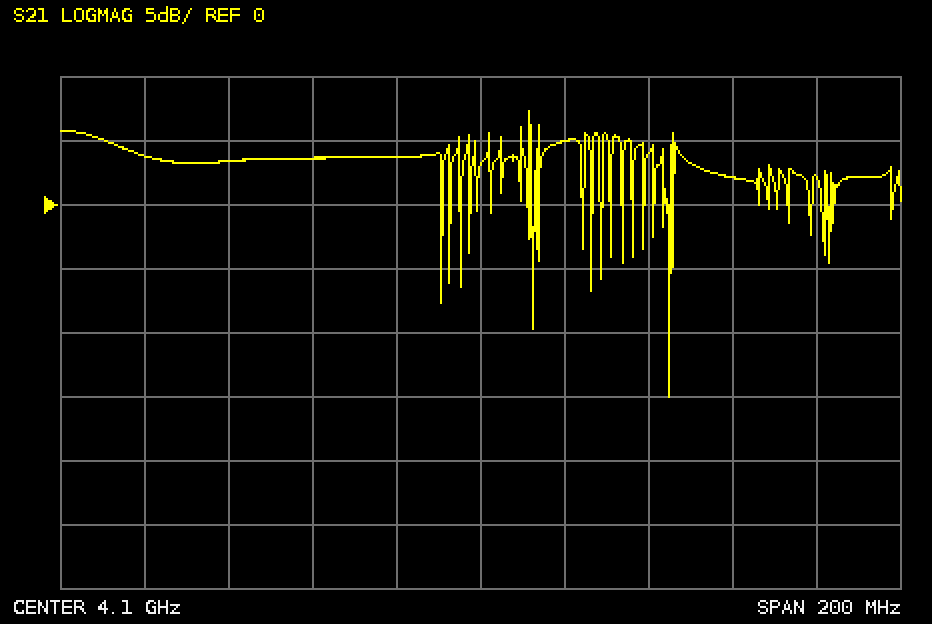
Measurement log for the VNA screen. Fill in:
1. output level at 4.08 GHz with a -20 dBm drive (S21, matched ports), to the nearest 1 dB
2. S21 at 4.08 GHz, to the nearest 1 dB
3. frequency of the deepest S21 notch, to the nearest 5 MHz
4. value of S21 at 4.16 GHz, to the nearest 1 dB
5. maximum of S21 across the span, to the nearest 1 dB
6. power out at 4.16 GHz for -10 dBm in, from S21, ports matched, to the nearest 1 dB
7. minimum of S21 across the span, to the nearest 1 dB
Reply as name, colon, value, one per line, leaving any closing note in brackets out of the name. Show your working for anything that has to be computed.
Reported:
output level at 4.08 GHz with a -20 dBm drive (S21, matched ports), to the nearest 1 dB: -20 dBm + (4 dB) = -16 dBm
S21 at 4.08 GHz, to the nearest 1 dB: 4 dB
frequency of the deepest S21 notch, to the nearest 5 MHz: 4.145 GHz
value of S21 at 4.16 GHz, to the nearest 1 dB: 2 dB
maximum of S21 across the span, to the nearest 1 dB: 7 dB
power out at 4.16 GHz for -10 dBm in, from S21, ports matched, to the nearest 1 dB: -10 dBm + (2 dB) = -8 dBm
minimum of S21 across the span, to the nearest 1 dB: -15 dB
